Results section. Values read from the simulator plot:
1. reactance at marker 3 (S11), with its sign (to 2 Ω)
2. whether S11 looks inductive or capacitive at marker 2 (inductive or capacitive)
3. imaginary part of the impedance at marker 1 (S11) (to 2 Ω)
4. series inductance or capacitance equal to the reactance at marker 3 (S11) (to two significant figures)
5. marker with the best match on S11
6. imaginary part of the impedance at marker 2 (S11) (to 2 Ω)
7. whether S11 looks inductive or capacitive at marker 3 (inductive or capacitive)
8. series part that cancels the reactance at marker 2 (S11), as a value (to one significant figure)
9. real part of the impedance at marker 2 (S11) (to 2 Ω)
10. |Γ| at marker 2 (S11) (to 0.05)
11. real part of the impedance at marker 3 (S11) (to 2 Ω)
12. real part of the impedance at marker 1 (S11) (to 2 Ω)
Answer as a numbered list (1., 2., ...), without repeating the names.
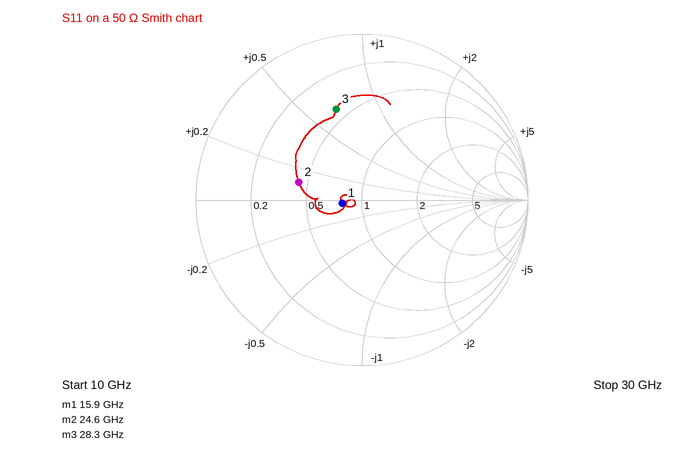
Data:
1. +34 Ω
2. inductive
3. -2 Ω
4. 190 pH
5. marker 1
6. +6 Ω
7. inductive
8. 1 pF
9. 22 Ω
10. 0.40
11. 20 Ω
12. 40 Ω
